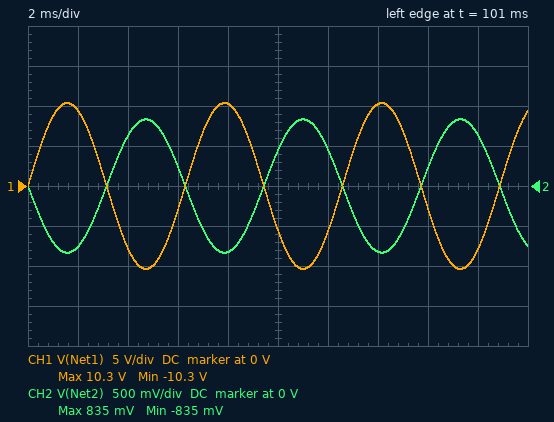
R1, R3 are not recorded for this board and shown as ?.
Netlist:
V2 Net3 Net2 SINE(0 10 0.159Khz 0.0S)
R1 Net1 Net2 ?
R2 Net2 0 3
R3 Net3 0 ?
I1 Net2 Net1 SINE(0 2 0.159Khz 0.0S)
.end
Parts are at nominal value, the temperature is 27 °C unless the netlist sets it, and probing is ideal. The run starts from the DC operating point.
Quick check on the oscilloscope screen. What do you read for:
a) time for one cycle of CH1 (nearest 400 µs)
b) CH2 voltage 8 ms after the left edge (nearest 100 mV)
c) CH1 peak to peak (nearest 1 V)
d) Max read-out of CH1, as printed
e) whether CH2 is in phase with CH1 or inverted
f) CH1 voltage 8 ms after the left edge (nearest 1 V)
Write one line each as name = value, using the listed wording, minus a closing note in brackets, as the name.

time for one cycle of CH1 = 6.4 ms
CH2 voltage 8 ms after the left edge = -800 mV
CH1 peak to peak = 21 V
Max read-out of CH1, as printed = 10.3 V
whether CH2 is in phase with CH1 or inverted = inverted
CH1 voltage 8 ms after the left edge = 10 V
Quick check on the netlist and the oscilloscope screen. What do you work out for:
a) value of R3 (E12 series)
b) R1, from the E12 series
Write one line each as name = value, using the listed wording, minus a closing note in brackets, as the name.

value of R3 = 33 Ω
R1, from the E12 series = 5.6 Ω
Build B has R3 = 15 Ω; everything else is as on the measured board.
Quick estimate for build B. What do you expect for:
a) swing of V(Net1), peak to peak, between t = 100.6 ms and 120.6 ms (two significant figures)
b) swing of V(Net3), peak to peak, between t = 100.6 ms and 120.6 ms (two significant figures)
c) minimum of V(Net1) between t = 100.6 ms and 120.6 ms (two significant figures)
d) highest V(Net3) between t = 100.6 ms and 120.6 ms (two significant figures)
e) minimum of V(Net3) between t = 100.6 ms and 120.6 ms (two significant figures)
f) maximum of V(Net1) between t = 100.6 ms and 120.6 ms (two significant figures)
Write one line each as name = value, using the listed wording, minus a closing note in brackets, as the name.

swing of V(Net1), peak to peak, between t = 100.6 ms and 120.6 ms = 19 V
swing of V(Net3), peak to peak, between t = 100.6 ms and 120.6 ms = 17 V
minimum of V(Net1) between t = 100.6 ms and 120.6 ms = -9.5 V
highest V(Net3) between t = 100.6 ms and 120.6 ms = 8.3 V
minimum of V(Net3) between t = 100.6 ms and 120.6 ms = -8.3 V
maximum of V(Net1) between t = 100.6 ms and 120.6 ms = 9.5 V
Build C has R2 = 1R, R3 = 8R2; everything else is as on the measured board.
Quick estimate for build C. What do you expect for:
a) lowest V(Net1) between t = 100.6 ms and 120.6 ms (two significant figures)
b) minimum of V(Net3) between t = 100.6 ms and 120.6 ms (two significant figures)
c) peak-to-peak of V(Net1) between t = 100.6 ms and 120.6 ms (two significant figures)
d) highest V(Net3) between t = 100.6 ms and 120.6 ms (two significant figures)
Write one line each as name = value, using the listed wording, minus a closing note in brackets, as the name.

lowest V(Net1) between t = 100.6 ms and 120.6 ms = -10 V
minimum of V(Net3) between t = 100.6 ms and 120.6 ms = -8.9 V
peak-to-peak of V(Net1) between t = 100.6 ms and 120.6 ms = 20 V
highest V(Net3) between t = 100.6 ms and 120.6 ms = 8.9 V
